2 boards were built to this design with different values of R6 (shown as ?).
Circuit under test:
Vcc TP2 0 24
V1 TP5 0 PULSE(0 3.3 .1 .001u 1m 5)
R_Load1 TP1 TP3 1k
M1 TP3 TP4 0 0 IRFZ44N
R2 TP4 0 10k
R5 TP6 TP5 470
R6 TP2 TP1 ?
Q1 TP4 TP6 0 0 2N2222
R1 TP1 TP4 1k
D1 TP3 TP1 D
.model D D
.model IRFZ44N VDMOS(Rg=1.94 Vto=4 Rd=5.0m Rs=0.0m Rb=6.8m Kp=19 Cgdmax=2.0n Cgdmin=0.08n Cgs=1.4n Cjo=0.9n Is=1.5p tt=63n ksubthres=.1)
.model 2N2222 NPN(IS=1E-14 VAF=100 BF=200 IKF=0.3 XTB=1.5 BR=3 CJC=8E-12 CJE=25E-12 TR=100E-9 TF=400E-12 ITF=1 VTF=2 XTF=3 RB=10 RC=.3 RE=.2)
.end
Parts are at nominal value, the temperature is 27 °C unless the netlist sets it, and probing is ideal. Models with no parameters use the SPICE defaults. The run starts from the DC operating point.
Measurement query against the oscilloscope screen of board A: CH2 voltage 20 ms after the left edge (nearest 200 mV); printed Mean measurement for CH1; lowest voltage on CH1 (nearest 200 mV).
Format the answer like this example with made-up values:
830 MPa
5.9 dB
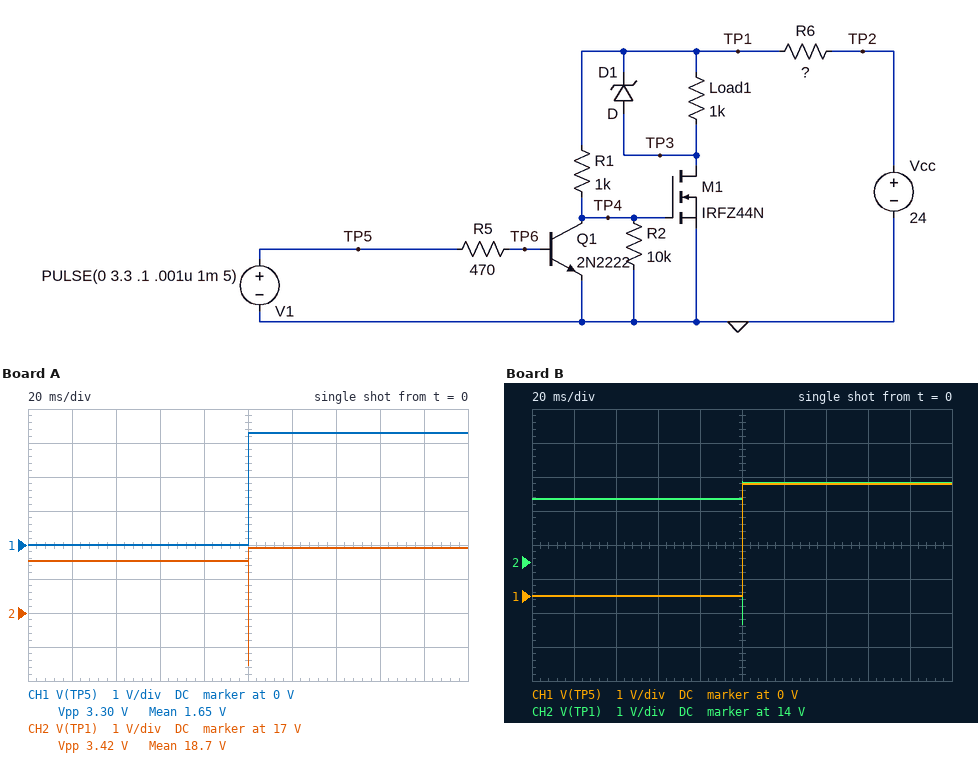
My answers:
18.6 V
1.65 V
0 V
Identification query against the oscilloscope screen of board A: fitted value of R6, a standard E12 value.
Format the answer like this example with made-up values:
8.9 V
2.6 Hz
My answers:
270 Ω
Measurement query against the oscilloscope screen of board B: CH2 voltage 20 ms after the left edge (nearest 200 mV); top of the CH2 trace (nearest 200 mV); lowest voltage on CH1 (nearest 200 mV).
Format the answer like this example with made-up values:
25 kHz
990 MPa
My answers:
15.8 V
16.4 V
0 V
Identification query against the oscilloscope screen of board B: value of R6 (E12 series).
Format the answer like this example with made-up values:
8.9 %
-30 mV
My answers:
470 Ω
